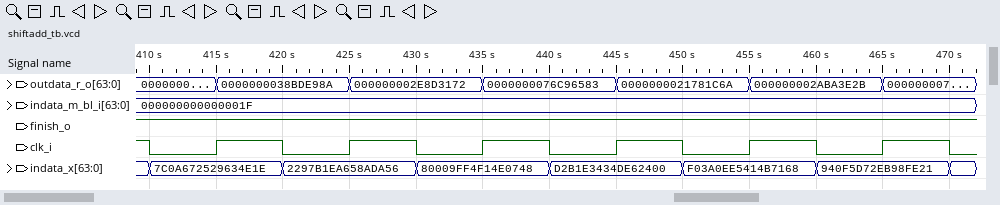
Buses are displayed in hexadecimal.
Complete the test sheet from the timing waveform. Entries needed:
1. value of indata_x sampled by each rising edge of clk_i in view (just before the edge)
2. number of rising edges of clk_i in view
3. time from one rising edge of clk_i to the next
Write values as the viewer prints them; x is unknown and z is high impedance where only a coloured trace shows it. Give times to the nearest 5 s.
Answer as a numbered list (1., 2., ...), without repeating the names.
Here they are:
1. 7C0A672529634E1E, 2297B1EA658ADA56, 80009FF4F14E0748, D2B1E3434DE62400, F03A0EE5414B7168, 940F5D72EB98FE21
2. 6
3. 10 s
